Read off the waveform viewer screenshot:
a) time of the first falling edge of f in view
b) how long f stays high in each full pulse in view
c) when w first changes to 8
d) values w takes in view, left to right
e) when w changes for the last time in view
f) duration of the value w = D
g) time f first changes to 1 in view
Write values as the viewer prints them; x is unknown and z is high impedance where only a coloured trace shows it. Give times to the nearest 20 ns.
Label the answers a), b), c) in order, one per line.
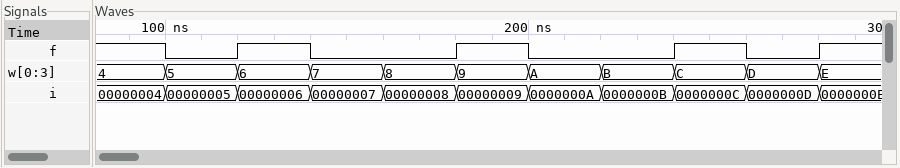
a) 100 ns
b) 20 ns, 20 ns, 20 ns
c) 160 ns
d) 4, 5, 6, 7, 8, 9, A, B, C, D, E
e) 280 ns
f) 20 ns
g) 120 ns
